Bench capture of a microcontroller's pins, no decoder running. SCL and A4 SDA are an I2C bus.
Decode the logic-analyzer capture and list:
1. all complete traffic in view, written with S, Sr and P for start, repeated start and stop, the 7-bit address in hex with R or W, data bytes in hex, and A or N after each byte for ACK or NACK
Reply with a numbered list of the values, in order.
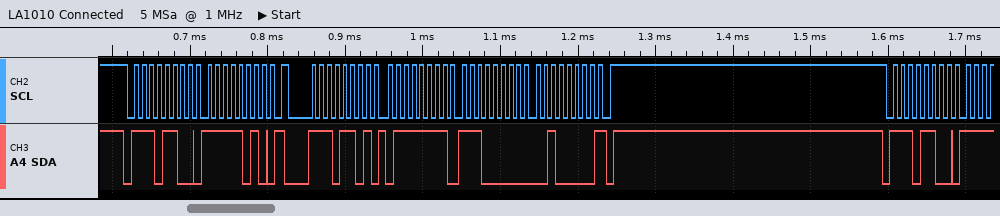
1. S 76W A FA A Sr 76R A 7F A E0 A 20 N P S 76W A
